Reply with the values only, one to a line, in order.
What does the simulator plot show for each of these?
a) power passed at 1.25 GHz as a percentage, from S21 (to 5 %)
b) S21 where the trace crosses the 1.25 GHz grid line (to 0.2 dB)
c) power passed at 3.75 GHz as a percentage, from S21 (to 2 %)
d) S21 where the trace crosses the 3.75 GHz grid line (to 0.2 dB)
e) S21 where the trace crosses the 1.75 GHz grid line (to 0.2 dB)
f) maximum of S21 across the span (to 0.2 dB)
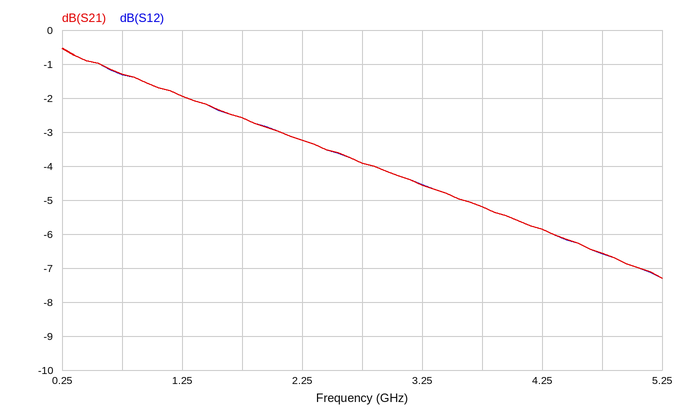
65 %
-2.0 dB
30 %
-5.2 dB
-2.6 dB
-0.6 dB
